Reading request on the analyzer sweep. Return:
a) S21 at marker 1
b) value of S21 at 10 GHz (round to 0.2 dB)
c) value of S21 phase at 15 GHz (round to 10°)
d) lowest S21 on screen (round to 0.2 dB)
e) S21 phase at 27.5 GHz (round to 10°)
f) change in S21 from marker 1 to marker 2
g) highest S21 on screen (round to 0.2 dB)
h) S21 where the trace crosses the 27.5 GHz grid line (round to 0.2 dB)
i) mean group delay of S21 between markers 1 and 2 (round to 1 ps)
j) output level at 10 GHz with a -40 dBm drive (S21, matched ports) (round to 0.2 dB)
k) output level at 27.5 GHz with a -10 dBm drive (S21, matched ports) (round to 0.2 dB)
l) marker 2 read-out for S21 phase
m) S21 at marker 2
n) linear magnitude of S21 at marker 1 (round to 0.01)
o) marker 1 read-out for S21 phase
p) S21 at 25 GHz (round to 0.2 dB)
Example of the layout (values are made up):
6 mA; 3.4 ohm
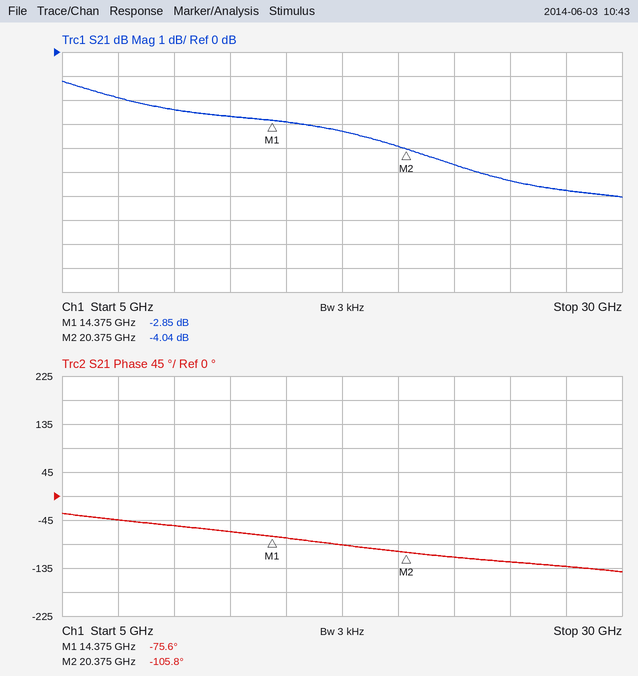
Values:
-2.85 dB; -2.4 dB; -80°; -6.0 dB; -130°; -1.19 dB; -1.2 dB; -5.8 dB; 14 ps; -42.4 dBm; -15.8 dBm; -105.8°; -4.04 dB; 0.72; -75.6°; -5.4 dB
